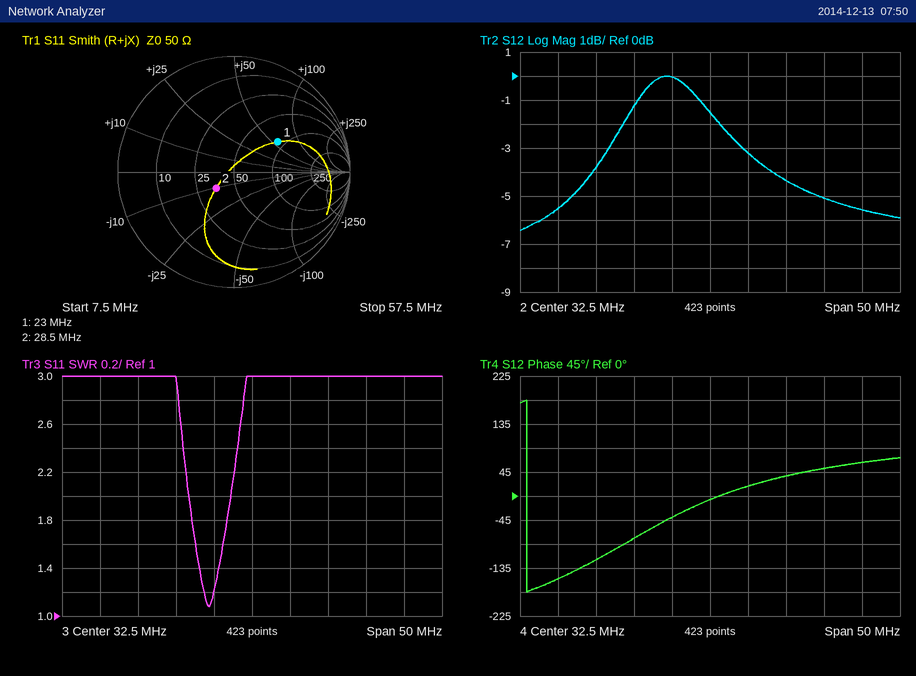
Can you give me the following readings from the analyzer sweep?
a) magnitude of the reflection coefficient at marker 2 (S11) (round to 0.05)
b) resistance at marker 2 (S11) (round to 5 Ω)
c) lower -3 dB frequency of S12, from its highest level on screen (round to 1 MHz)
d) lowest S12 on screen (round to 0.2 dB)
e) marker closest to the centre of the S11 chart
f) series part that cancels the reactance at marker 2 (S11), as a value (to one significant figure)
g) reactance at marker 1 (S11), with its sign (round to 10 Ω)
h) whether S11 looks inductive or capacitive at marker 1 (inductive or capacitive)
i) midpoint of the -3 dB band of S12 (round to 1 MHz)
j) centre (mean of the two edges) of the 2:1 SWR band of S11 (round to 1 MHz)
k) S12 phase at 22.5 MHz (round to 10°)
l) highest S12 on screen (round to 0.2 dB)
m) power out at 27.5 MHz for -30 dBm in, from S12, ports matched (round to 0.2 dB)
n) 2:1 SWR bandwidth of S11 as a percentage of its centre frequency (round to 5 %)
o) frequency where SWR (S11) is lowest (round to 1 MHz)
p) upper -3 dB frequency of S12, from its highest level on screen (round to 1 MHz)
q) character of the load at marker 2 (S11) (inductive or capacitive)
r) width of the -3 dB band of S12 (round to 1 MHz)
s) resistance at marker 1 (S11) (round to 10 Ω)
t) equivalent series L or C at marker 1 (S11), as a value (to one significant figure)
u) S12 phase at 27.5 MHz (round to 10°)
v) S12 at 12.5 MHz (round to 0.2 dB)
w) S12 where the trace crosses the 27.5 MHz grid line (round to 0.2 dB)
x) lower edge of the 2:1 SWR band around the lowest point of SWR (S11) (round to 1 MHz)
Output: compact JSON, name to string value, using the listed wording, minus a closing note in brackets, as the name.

{"magnitude of the reflection coefficient at marker 2 (S11)": "0.20", "resistance at marker 2 (S11)": "35 Ω", "lower -3 dB frequency of S12, from its highest level on screen": "19 MHz", "lowest S12 on screen": "-6.4 dB", "marker closest to the centre of the S11 chart": "marker 2", "series part that cancels the reactance at marker 2 (S11), as a value": "60 nH", "reactance at marker 1 (S11), with its sign": "+60 Ω", "whether S11 looks inductive or capacitive at marker 1": "inductive", "midpoint of the -3 dB band of S12": "28 MHz", "centre (mean of the two edges) of the 2:1 SWR band of S11": "27 MHz", "S12 phase at 22.5 MHz": "-80°", "highest S12 on screen": "0.0 dB", "power out at 27.5 MHz for -30 dBm in, from S12, ports matched": "-30.0 dBm", "2:1 SWR bandwidth of S11 as a percentage of its centre frequency": "20 %", "frequency where SWR (S11) is lowest": "27 MHz", "upper -3 dB frequency of S12, from its highest level on screen": "37 MHz", "character of the load at marker 2 (S11)": "capacitive", "width of the -3 dB band of S12": "18 MHz", "resistance at marker 1 (S11)": "90 Ω", "equivalent series L or C at marker 1 (S11), as a value": "400 nH", "S12 phase at 27.5 MHz": "-40°", "S12 at 12.5 MHz": "-5.6 dB", "S12 where the trace crosses the 27.5 MHz grid line": "0.0 dB", "lower edge of the 2:1 SWR band around the lowest point of SWR (S11)": "24 MHz"}
